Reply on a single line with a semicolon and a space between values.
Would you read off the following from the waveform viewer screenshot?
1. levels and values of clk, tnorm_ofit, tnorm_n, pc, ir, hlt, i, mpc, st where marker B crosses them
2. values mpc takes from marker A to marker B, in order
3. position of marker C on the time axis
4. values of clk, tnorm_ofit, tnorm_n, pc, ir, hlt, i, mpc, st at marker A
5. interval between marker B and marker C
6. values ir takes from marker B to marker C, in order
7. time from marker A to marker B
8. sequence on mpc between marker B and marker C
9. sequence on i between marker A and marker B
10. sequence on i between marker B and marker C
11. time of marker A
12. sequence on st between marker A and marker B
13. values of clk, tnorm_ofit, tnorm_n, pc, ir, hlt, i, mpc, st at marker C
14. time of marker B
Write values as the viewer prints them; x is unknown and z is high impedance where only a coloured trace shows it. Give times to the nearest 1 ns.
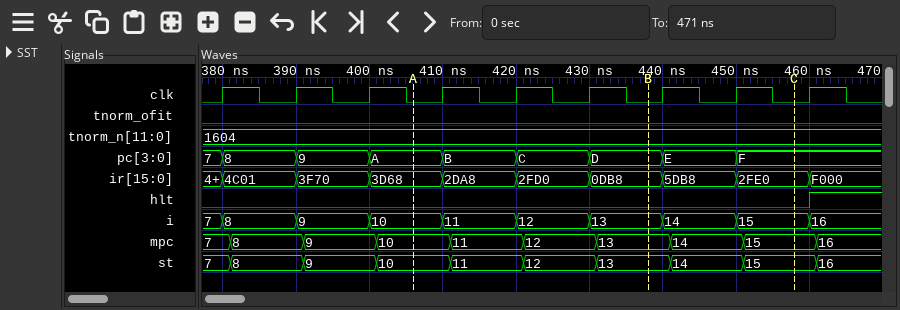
clk=0, tnorm_ofit=0, tnorm_n=1604, pc=D, ir=0DB8, hlt=0, i=13, mpc=13, st=13; 10, 11, 12, 13; 458 ns; clk=0, tnorm_ofit=0, tnorm_n=1604, pc=A, ir=3D68, hlt=0, i=10, mpc=10, st=10; 20 ns; 0DB8, 5DB8, 2FE0; 32 ns; 13, 14, 15; 10, 11, 12, 13; 13, 14, 15; 406 ns; 10, 11, 12, 13; clk=0, tnorm_ofit=0, tnorm_n=1604, pc=F, ir=2FE0, hlt=0, i=15, mpc=15, st=15; 438 ns
